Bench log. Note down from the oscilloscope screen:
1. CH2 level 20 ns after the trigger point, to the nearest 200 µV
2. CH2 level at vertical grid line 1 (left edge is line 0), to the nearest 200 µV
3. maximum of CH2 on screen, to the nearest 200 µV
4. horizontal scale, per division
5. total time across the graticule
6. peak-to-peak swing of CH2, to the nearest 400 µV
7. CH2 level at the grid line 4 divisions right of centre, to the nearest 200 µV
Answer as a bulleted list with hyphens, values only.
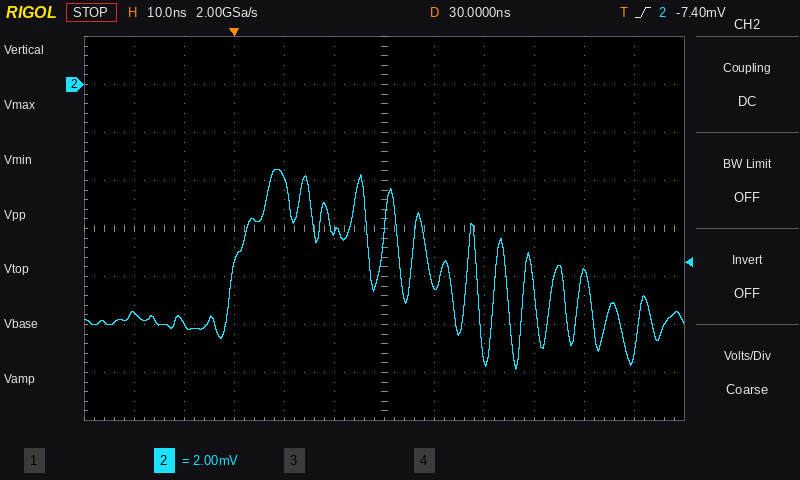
- -6.2 mV
- -9.6 mV
- -3.6 mV
- 10 ns
- 120 ns
- 8.4 mV
- -7.8 mV
